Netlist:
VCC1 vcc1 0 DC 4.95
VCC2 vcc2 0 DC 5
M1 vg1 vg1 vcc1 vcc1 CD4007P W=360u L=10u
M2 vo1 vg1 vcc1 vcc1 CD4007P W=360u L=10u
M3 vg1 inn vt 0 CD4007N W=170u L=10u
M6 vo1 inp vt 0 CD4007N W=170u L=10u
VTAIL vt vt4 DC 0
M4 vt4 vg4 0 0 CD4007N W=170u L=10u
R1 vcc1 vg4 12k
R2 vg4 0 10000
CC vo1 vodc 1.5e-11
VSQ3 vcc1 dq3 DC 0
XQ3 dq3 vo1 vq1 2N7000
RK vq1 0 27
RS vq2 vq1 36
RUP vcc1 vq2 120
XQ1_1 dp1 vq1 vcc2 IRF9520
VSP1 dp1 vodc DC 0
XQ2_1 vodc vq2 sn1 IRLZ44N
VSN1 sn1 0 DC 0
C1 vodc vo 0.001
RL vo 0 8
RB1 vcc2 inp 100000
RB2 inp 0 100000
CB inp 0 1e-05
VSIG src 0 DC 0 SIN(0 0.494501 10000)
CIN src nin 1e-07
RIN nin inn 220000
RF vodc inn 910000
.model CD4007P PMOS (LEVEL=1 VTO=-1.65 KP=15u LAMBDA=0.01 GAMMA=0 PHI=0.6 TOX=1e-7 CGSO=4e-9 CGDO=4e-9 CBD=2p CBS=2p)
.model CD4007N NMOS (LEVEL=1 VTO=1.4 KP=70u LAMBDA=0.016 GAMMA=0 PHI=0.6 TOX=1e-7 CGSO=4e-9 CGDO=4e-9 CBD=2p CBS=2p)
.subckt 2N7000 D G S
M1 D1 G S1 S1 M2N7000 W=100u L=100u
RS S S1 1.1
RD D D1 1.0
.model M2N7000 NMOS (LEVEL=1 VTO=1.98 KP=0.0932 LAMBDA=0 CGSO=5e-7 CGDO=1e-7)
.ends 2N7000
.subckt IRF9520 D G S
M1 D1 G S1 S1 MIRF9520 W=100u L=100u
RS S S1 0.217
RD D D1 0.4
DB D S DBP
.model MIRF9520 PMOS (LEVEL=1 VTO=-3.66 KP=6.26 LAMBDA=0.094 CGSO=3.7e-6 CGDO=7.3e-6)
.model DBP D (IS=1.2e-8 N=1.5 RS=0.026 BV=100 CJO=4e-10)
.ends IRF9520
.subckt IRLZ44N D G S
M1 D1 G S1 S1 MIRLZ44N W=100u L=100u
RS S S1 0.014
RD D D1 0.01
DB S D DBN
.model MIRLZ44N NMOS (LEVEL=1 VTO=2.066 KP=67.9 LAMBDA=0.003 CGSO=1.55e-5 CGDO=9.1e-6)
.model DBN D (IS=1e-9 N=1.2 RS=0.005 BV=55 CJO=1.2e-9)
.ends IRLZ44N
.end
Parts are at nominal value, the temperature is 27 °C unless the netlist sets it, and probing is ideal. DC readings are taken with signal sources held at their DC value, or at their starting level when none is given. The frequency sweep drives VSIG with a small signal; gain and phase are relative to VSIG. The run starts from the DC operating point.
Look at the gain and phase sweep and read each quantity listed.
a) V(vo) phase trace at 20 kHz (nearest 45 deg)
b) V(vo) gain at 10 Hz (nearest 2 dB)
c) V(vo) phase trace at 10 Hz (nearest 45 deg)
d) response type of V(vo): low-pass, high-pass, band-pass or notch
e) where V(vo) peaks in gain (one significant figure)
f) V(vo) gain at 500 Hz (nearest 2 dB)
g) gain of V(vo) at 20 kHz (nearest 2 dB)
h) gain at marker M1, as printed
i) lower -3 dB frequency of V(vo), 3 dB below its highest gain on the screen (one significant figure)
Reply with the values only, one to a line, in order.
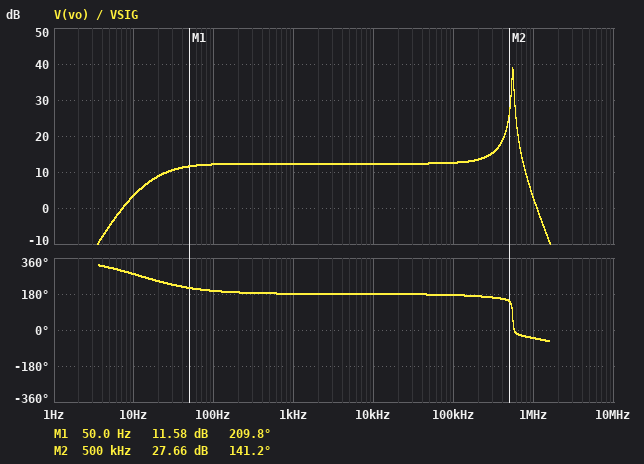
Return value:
180 deg
4 dB
270 deg
band-pass
500 kHz
12 dB
12 dB
11.58 dB
500 kHz
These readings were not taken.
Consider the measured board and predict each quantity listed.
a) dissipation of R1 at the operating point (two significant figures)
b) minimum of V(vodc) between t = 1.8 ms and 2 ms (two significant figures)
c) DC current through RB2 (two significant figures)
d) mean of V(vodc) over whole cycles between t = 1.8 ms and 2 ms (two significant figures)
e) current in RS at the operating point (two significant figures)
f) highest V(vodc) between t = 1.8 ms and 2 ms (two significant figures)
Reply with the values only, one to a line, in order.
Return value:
610 µW
460 mV
25 µA
2.5 V
24 mA
4.5 V
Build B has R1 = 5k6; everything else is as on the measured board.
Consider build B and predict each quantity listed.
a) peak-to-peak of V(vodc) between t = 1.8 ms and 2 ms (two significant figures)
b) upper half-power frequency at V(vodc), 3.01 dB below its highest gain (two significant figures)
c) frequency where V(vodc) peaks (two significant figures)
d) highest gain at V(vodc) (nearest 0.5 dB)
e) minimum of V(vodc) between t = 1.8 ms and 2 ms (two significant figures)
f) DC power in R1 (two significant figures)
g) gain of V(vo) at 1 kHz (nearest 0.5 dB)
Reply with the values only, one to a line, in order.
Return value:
4.0 V
590 kHz
560 kHz
30.5 dB
560 mV
560 µW
12.0 dB
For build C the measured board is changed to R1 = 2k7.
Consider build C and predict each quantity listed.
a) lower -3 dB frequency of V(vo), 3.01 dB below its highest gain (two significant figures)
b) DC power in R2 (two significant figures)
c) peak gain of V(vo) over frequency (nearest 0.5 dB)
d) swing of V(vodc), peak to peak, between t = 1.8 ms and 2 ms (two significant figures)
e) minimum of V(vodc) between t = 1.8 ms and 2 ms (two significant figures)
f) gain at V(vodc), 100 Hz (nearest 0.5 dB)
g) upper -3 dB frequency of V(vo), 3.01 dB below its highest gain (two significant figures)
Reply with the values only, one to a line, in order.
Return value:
460 kHz
1.5 mW
23.0 dB
3.9 V
630 mV
11.5 dB
600 kHz
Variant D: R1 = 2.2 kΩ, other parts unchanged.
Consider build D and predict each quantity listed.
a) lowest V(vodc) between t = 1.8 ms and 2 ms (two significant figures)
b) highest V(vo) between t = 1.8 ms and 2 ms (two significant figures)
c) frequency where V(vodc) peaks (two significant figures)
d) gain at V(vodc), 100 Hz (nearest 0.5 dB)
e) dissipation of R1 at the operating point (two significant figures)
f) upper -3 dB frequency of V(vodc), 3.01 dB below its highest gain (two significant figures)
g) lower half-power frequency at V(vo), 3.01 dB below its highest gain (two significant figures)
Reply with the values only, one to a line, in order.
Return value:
640 mV
1.9 V
530 kHz
11.5 dB
360 µW
600 kHz
450 kHz
